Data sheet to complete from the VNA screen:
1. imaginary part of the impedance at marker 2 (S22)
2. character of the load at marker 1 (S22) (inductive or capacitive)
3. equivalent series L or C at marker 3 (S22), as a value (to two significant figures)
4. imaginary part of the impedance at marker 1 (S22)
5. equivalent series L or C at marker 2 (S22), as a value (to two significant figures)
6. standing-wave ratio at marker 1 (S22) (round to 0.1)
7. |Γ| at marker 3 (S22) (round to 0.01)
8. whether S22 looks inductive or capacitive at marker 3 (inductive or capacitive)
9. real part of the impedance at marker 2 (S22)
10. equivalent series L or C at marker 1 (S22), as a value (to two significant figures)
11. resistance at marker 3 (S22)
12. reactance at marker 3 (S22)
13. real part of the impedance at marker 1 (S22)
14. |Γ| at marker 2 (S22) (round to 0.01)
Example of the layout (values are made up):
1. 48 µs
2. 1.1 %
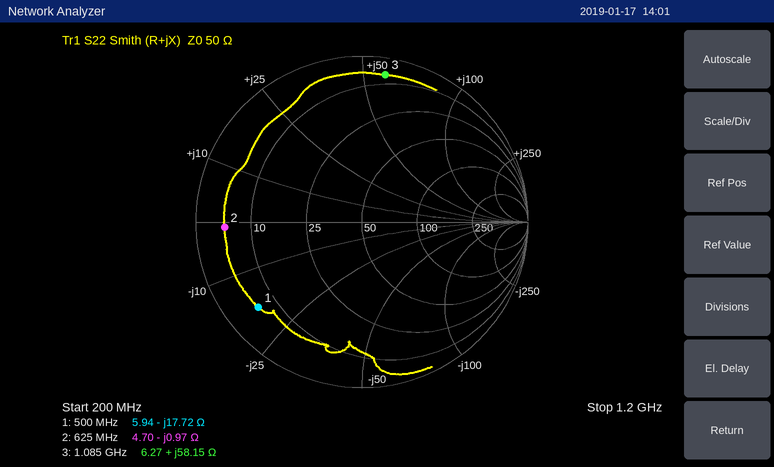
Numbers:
1. -0.97 Ω
2. capacitive
3. 8.5 nH
4. -17.72 Ω
5. 260 pF
6. 9.5
7. 0.90
8. inductive
9. 4.70 Ω
10. 18 pF
11. 6.27 Ω
12. +58.15 Ω
13. 5.94 Ω
14. 0.83
